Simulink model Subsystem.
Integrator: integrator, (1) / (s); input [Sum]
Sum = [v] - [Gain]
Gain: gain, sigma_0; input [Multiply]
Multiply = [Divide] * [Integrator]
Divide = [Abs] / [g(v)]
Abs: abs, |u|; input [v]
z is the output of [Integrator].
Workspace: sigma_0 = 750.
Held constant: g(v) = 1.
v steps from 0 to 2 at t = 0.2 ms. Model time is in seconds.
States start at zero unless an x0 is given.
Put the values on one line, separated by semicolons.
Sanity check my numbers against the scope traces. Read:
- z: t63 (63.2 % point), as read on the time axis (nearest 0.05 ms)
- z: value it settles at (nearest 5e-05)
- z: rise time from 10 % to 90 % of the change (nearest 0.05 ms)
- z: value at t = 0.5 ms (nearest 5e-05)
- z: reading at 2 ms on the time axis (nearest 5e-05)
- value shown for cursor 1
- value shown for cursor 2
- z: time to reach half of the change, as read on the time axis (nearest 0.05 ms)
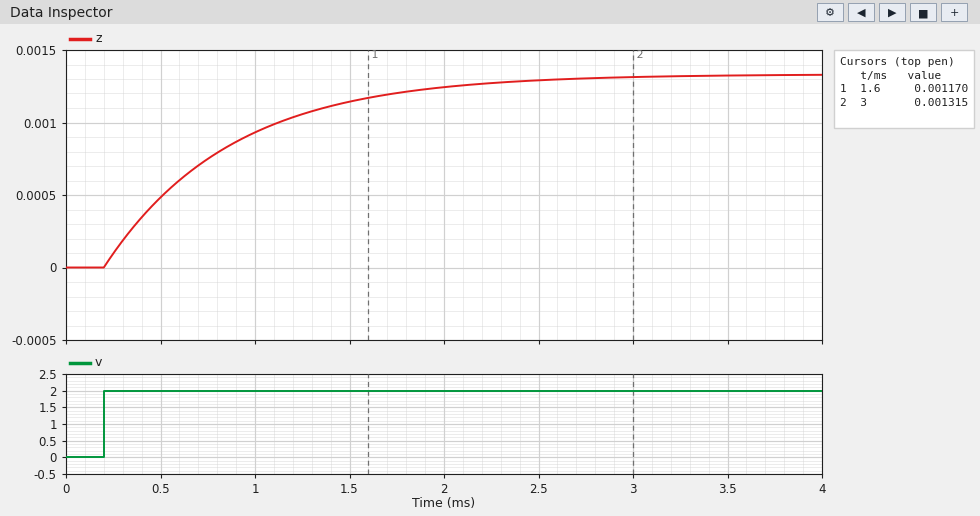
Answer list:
0.85 ms; 0.00135; 1.45 ms; 0.00050; 0.00125; 0.001170; 0.001315; 0.65 ms
